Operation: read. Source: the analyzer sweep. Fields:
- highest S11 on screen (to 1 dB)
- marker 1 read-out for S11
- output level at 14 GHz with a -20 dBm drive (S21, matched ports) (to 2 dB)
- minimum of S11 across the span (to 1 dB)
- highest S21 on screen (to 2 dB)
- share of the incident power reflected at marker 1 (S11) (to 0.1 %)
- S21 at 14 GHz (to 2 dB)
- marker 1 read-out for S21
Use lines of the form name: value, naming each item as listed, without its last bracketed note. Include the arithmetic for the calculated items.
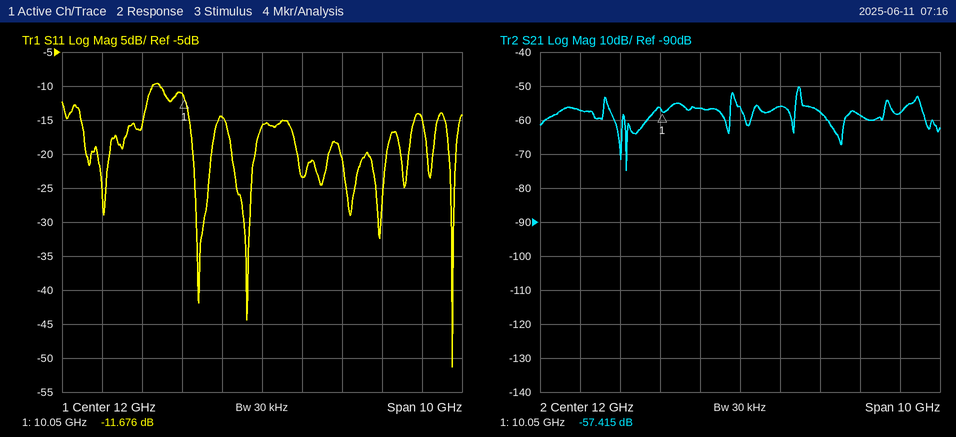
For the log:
highest S11 on screen: -10 dB
marker 1 read-out for S11: -11.676 dB
output level at 14 GHz with a -20 dBm drive (S21, matched ports): -20 dBm + (-58 dB) = -78 dBm
minimum of S11 across the span: -51 dB
highest S21 on screen: -50 dB
share of the incident power reflected at marker 1 (S11): 10^(-11.676/10) ≈ 6.8 %
S21 at 14 GHz: -58 dB
marker 1 read-out for S21: -57.415 dB
